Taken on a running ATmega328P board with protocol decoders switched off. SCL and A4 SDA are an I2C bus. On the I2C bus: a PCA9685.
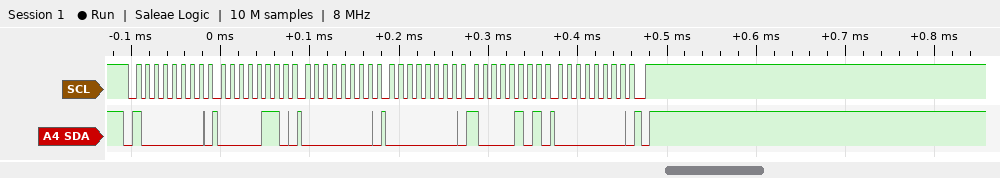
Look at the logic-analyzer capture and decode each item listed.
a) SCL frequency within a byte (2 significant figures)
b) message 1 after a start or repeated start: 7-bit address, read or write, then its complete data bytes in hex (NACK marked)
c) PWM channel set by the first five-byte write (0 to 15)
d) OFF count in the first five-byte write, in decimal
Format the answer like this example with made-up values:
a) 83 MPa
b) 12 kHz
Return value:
a) 100 kHz
b) 0x40 write: 06 00 00 85 00
c) 0
d) 133
